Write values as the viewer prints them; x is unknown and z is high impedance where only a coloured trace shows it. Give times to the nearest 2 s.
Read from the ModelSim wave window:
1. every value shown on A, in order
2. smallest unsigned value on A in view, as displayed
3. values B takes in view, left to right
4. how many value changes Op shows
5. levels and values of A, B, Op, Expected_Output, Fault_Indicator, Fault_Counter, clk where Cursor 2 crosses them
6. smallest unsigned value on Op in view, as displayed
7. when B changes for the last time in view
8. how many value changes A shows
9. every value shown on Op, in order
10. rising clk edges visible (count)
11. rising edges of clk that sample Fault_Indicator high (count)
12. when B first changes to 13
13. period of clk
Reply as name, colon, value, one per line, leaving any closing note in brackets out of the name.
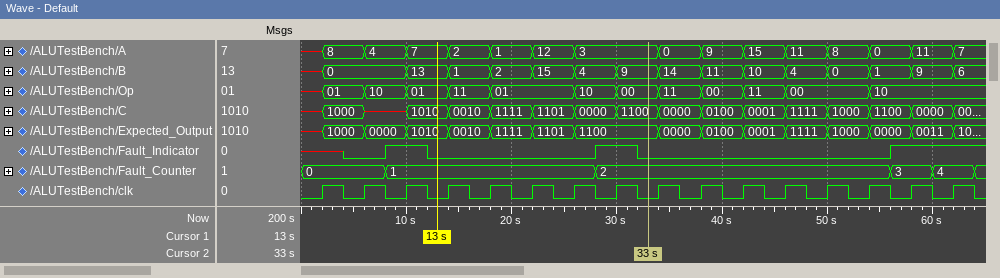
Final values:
every value shown on A, in order: x, 8, 4, 7, 2, 1, 12, 3, 0, 9, 15, 11, 8, 0, 11, 7
smallest unsigned value on A in view, as displayed: 0
values B takes in view, left to right: x, 0, 13, 1, 2, 15, 4, 9, 14, 11, 10, 4, 0, 1, 9, 6
how many value changes Op shows: 12
levels and values of A, B, Op, Expected_Output, Fault_Indicator, Fault_Counter, clk where Cursor 2 crosses them: A=3, B=9, Op=00, Expected_Output=1100, Fault_Indicator=0, Fault_Counter=2, clk=0
smallest unsigned value on Op in view, as displayed: 00
when B changes for the last time in view: 62 s
how many value changes A shows: 15
every value shown on Op, in order: x, 01, 10, 01, 11, 01, 10, 00, 11, 00, 11, 00, 10
rising clk edges visible: 16
rising edges of clk that sample Fault_Indicator high: 4
when B first changes to 13: 10 s
period of clk: 4 s
